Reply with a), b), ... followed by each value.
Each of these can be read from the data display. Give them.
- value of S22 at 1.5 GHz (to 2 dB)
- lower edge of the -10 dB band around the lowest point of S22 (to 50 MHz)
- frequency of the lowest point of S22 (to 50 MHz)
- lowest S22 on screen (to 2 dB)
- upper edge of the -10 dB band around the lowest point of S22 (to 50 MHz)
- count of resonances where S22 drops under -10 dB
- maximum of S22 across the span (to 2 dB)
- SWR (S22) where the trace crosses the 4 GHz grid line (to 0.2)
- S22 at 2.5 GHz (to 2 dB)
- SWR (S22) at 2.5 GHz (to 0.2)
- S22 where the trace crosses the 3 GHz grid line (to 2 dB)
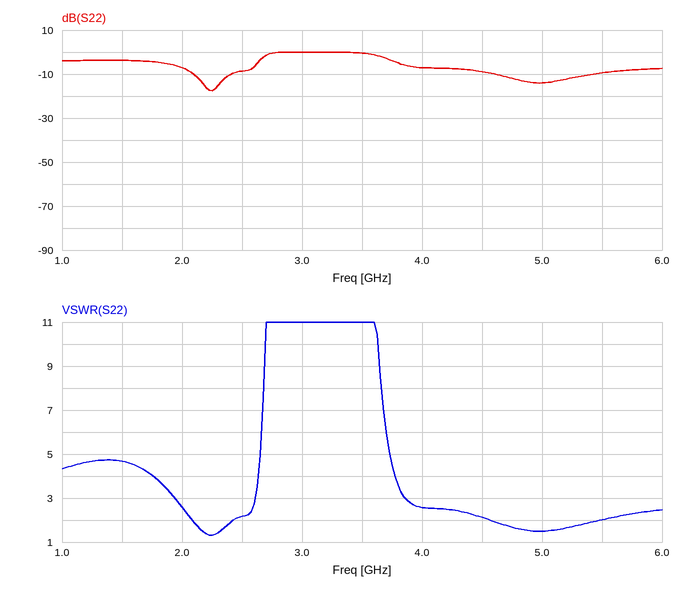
a) -4 dB
b) 2.10 GHz
c) 2.25 GHz
d) -18 dB
e) 2.40 GHz
f) 2
g) 0 dB
h) 2.6
i) -8 dB
j) 2.2
k) 0 dB
